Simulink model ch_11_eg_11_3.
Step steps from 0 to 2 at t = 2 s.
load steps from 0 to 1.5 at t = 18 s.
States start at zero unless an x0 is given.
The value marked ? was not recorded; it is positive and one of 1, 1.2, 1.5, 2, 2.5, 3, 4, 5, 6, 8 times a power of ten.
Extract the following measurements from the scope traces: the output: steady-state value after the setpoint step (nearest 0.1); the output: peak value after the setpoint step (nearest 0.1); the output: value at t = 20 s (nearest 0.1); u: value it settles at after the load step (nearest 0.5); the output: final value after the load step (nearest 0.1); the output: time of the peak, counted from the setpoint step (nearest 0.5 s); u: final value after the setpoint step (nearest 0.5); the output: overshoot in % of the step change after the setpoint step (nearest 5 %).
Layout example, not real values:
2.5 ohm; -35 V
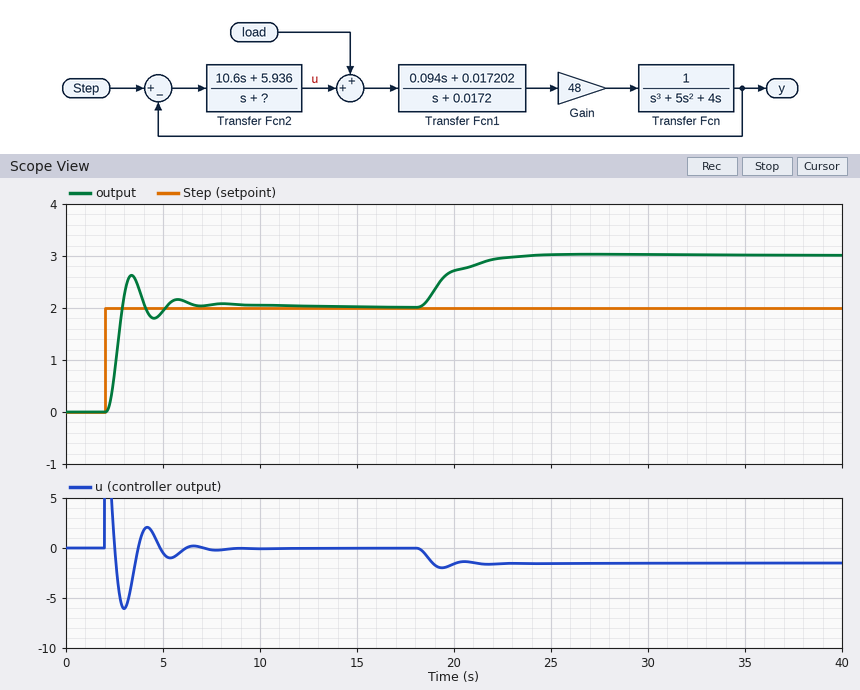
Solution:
2.0; 2.6; 2.7; -1.5; 3.0; 1.5 s; 0.0; 30 %
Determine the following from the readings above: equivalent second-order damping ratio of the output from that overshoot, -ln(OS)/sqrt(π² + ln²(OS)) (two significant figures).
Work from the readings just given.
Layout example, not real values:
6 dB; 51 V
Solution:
0.36
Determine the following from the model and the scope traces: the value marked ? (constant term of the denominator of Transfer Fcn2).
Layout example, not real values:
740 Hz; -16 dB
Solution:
4
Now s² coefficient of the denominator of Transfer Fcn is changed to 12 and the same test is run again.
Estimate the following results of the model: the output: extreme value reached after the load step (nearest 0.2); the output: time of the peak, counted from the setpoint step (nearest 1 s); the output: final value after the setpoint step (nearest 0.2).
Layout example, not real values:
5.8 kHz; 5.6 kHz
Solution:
3.0; 3 s; 2.0
